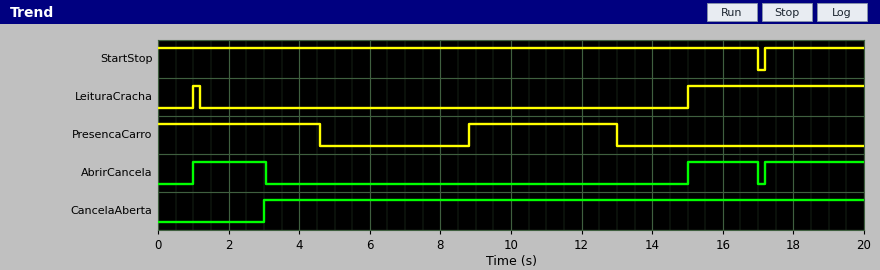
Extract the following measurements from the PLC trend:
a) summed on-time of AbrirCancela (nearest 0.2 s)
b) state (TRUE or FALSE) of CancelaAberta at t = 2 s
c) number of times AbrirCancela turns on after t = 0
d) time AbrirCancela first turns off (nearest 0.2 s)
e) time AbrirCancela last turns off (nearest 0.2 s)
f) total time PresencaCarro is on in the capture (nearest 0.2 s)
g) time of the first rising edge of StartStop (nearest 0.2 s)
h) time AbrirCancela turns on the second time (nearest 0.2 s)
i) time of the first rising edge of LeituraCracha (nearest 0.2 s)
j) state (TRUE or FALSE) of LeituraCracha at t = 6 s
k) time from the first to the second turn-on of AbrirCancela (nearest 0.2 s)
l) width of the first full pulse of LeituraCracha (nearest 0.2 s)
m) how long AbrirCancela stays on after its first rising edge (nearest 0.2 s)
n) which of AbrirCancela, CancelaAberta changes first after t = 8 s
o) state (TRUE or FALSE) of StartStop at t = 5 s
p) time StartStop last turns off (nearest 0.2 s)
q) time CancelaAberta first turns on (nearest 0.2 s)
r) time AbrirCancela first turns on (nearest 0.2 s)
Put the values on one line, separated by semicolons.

6.8 s; FALSE; 3; 3.0 s; 17.0 s; 8.8 s; 17.2 s; 15.0 s; 1.0 s; FALSE; 14.0 s; 0.2 s; 2.0 s; AbrirCancela; TRUE; 17.0 s; 3.0 s; 1.0 s
